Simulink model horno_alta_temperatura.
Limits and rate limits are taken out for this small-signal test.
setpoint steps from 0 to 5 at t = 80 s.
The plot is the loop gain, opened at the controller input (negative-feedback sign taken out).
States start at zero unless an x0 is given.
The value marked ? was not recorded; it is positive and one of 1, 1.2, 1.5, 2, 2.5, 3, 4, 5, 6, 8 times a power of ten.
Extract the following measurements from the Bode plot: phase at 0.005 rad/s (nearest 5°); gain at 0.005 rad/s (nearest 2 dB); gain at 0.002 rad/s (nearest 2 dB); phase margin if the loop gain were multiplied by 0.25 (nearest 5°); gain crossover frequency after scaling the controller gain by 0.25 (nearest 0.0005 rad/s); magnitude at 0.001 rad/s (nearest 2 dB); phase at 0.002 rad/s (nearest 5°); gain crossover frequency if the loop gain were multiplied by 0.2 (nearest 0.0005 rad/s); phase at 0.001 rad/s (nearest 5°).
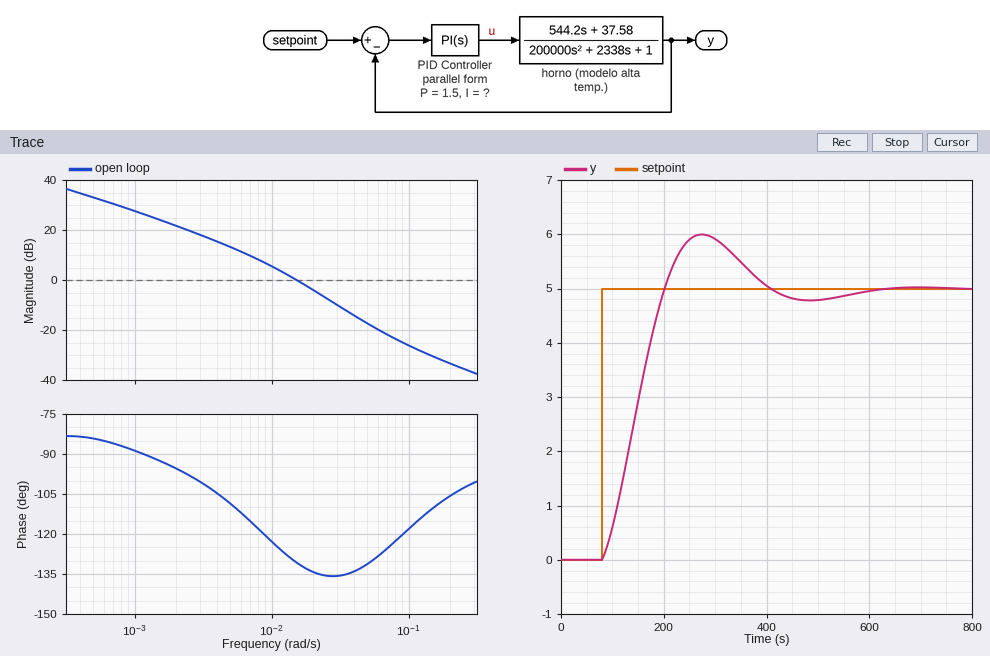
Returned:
-110°
14 dB
22 dB
70°
0.0055 rad/s
28 dB
-95°
0.0045 rad/s
-90°
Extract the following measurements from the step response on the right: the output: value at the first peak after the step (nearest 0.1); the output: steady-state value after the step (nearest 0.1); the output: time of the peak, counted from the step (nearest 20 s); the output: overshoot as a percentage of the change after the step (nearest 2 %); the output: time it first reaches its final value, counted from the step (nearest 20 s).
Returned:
6.0
5.0
200 s
20 %
120 s
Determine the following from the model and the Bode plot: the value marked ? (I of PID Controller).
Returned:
0.0005
